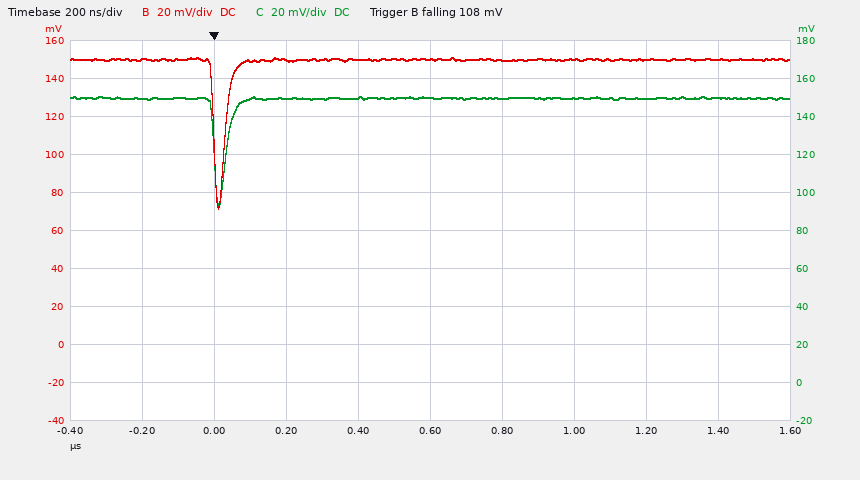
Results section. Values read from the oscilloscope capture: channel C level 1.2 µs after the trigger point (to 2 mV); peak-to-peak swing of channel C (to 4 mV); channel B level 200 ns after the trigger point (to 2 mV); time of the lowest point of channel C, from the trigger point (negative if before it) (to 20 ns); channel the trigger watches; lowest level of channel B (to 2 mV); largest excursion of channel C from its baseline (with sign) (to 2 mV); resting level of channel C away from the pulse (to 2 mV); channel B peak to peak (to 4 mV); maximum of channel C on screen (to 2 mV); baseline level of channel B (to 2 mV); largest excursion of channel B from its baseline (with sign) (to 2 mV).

150 mV
56 mV
150 mV
+20 ns
channel B
72 mV
-56 mV
150 mV
80 mV
150 mV
150 mV
-78 mV
